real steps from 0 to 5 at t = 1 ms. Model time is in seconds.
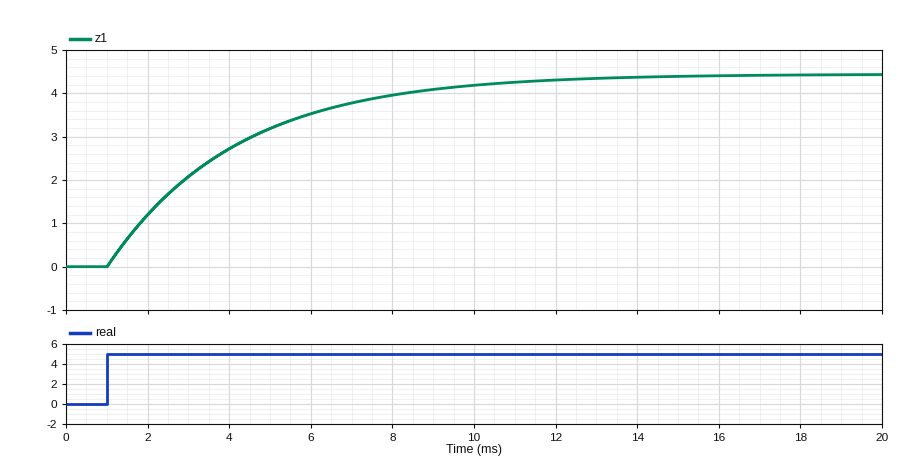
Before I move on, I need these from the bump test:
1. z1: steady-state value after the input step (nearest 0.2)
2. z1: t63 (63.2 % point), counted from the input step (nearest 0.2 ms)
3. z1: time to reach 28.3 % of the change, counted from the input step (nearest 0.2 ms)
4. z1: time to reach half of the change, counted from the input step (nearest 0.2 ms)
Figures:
4.4
3.2 ms
1.0 ms
2.2 ms
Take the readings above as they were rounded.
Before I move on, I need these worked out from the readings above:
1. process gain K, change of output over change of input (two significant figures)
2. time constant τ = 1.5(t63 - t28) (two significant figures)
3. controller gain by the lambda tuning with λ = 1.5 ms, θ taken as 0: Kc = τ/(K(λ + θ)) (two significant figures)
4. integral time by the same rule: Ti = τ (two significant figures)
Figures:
0.88
3.3 ms
2.5
3.3 ms
